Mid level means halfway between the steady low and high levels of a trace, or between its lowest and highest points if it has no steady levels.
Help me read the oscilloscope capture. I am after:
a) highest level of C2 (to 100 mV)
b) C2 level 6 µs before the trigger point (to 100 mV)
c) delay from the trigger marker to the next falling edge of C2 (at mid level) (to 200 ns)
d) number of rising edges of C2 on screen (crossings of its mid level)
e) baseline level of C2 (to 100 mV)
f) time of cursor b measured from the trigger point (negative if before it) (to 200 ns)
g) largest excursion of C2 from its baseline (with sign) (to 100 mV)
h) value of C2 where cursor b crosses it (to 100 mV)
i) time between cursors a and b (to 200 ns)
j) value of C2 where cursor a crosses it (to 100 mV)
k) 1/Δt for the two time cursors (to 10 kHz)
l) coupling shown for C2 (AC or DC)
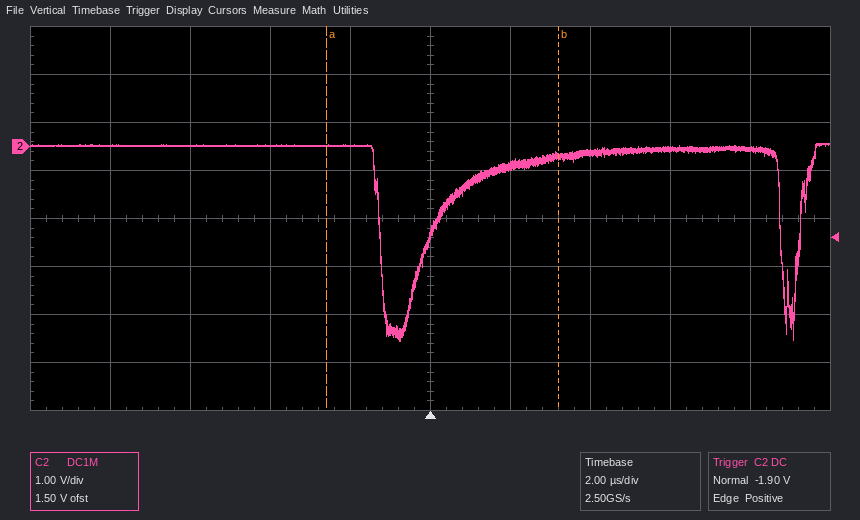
100 mV
0.0 V
8.8 µs
2
0.0 V
+3.2 µs
-4.1 V
-200 mV
5.8 µs
0.0 V
170 kHz
DC
